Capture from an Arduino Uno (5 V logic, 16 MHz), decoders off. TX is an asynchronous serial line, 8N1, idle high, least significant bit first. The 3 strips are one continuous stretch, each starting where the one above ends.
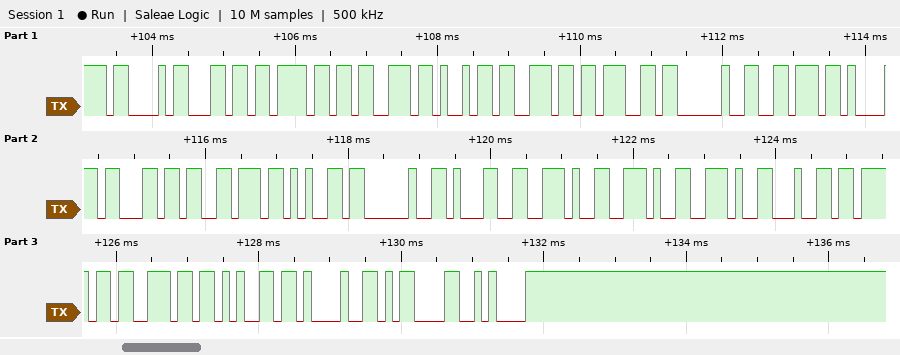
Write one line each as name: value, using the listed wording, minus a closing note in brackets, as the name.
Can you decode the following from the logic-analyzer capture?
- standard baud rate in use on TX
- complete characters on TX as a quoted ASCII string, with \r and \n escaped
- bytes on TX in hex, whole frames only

standard baud rate in use on TX: 9600 baud
complete characters on TX as a quoted ASCII string, with \r and \n escaped: "Closing valve 1...done!\r\n"
bytes on TX in hex, whole frames only: 43 6C 6F 73 69 6E 67 20 76 61 6C 76 65 20 31 2E 2E 2E 64 6F 6E 65 21 0D 0A
